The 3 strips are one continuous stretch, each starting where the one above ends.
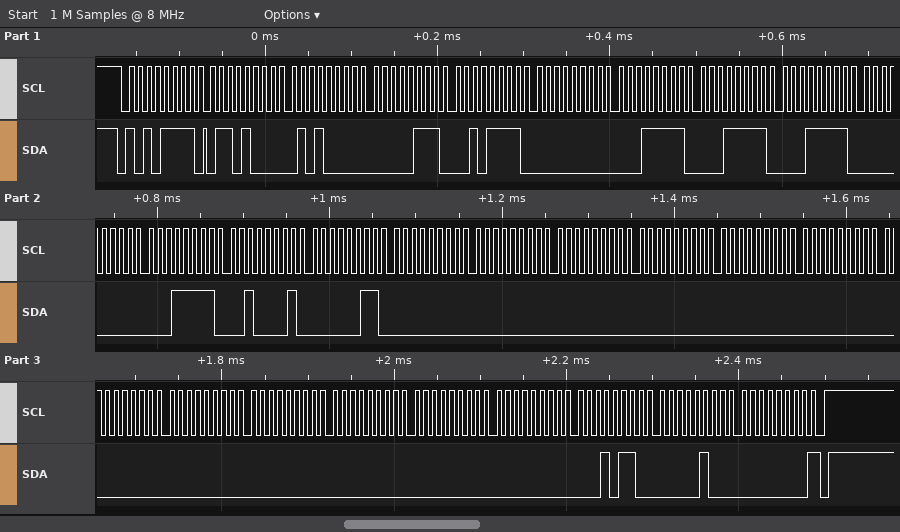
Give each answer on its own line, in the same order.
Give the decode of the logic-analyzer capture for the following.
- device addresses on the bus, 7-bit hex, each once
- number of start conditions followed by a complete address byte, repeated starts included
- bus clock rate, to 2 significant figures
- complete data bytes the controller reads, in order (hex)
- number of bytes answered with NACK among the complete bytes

0x57
1
100 kHz
68 50 07 2F 00 1F 1F 1F 00 1F 21 03 00 00 00 00 00 00 00 00 00 00 00 00 16 04 00
1
